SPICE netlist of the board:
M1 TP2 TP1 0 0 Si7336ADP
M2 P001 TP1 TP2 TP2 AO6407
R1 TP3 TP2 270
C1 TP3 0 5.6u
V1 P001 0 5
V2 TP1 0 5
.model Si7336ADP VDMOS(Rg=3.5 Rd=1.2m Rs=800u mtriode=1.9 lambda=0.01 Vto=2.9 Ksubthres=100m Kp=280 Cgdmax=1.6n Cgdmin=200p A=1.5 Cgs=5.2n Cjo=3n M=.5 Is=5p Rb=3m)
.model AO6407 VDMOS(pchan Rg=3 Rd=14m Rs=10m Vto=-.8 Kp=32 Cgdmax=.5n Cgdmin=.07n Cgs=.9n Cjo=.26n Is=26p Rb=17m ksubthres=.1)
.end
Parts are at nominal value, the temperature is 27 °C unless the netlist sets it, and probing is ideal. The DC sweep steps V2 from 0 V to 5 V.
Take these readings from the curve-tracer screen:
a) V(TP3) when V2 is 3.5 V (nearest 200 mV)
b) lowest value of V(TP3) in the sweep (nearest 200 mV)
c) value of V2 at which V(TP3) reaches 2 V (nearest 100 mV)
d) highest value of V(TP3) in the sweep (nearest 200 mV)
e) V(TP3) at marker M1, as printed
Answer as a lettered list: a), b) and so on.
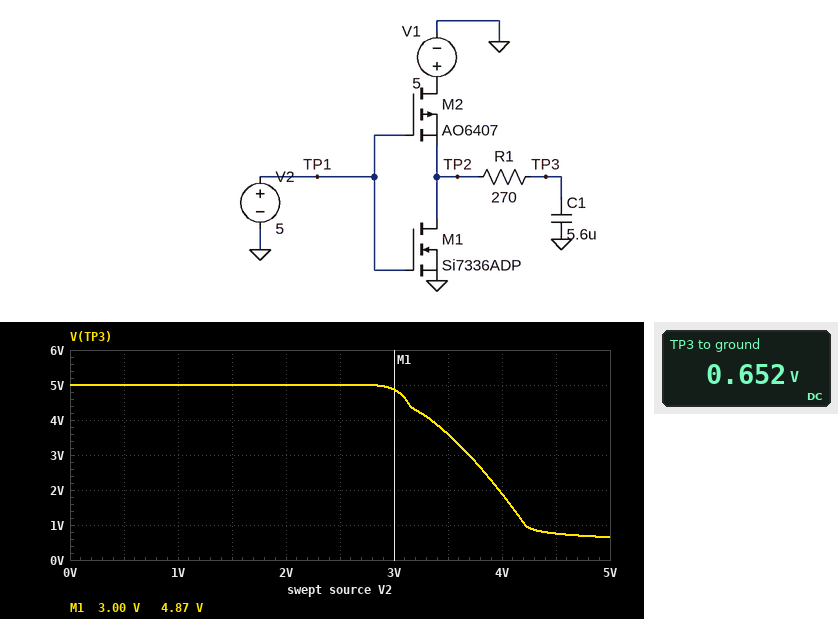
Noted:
a) 3.6 V
b) 600 mV
c) 4.0 V
d) 5.0 V
e) 4.87 V
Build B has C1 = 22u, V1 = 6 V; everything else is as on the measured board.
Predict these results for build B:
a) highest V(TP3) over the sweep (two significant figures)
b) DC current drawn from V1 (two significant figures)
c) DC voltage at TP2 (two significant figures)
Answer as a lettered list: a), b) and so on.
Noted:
a) 6.0 V
b) 260 A
c) 820 mV
